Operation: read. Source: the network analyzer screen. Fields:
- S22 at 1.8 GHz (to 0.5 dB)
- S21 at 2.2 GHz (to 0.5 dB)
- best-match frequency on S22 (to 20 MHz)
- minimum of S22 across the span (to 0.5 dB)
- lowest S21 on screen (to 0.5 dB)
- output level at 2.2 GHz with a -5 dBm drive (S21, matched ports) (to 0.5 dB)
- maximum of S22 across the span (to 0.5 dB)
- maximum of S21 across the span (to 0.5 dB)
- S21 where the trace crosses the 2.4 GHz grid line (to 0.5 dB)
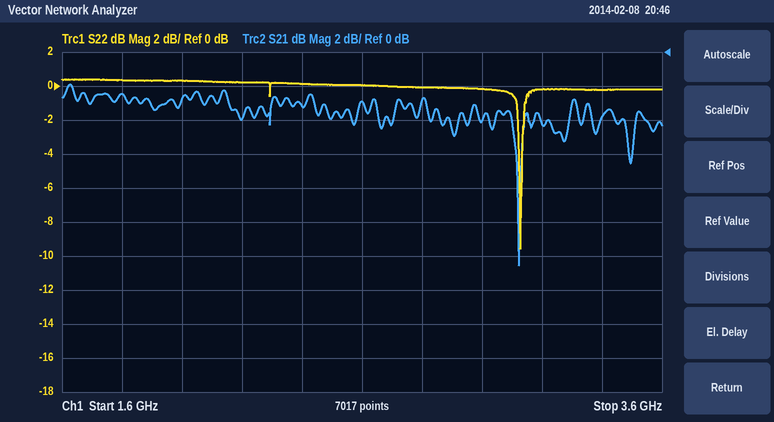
0.5 dB
-4.0 dB
3.12 GHz
-9.5 dB
-12.5 dB
-9.0 dBm
0.5 dB
-2.0 dB
-3.0 dB
